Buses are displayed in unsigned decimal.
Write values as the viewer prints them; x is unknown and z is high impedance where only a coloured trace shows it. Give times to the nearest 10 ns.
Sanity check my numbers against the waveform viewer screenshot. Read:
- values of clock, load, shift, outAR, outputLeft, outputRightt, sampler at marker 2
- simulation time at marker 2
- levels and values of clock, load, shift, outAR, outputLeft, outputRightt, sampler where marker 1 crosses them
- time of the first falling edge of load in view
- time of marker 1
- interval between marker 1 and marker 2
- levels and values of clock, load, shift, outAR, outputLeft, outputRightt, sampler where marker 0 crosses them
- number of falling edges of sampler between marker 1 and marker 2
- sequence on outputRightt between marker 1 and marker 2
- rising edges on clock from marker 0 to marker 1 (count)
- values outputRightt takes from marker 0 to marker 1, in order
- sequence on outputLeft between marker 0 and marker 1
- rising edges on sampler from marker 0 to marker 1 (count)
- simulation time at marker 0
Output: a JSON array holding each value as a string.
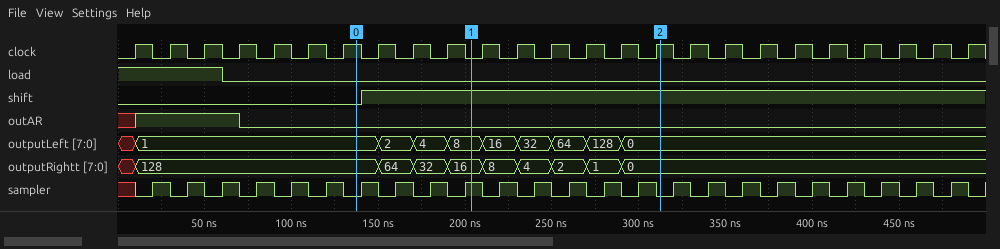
["clock=1, load=0, shift=1, outAR=0, outputLeft=0, outputRightt=0, sampler=0", "310 ns", "clock=0, load=0, shift=1, outAR=0, outputLeft=8, outputRightt=16, sampler=1", "60 ns", "200 ns", "110 ns", "clock=1, load=0, shift=0, outAR=0, outputLeft=1, outputRightt=128, sampler=0", "6", "16, 8, 4, 2, 1, 0", "3", "128, 64, 32, 16", "1, 2, 4, 8", "4", "140 ns"]
